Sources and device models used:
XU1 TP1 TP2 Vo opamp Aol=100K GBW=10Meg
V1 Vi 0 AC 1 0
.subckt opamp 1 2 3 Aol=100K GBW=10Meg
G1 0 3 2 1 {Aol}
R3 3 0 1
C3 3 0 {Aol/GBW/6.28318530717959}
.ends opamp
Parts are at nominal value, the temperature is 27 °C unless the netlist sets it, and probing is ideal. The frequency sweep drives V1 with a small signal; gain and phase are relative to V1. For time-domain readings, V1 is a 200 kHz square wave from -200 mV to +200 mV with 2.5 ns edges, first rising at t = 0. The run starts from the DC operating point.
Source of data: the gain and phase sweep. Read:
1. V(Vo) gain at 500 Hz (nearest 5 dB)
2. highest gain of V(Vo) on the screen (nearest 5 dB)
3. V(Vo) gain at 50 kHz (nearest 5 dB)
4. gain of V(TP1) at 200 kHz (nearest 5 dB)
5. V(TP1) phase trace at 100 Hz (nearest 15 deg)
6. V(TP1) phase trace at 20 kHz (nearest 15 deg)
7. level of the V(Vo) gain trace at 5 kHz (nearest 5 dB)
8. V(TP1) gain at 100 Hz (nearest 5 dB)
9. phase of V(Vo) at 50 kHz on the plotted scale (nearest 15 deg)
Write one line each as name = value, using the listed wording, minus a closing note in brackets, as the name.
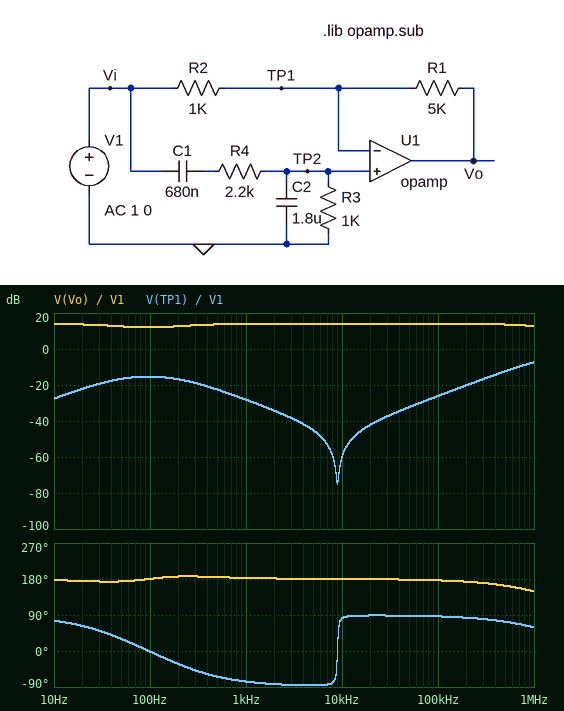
V(Vo) gain at 500 Hz = 15 dB
highest gain of V(Vo) on the screen = 15 dB
V(Vo) gain at 50 kHz = 15 dB
gain of V(TP1) at 200 kHz = -20 dB
V(TP1) phase trace at 100 Hz = 0 deg
V(TP1) phase trace at 20 kHz = 90 deg
level of the V(Vo) gain trace at 5 kHz = 15 dB
V(TP1) gain at 100 Hz = -15 dB
phase of V(Vo) at 50 kHz on the plotted scale = 180 deg
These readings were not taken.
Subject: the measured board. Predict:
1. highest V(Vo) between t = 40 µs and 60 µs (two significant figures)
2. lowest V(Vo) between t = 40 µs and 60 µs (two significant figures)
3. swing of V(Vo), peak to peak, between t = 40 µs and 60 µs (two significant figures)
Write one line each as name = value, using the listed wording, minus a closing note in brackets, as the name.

highest V(Vo) between t = 40 µs and 60 µs = 1.0 V
lowest V(Vo) between t = 40 µs and 60 µs = -990 mV
swing of V(Vo), peak to peak, between t = 40 µs and 60 µs = 2.0 V
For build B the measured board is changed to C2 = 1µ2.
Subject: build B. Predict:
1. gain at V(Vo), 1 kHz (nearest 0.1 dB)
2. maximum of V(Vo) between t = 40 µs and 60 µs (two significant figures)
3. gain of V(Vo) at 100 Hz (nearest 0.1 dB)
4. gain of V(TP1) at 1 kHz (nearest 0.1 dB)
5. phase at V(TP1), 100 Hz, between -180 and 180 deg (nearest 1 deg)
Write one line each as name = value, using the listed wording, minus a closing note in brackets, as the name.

gain at V(Vo), 1 kHz = 13.8 dB
maximum of V(Vo) between t = 40 µs and 60 µs = 1.0 V
gain of V(Vo) at 100 Hz = 11.6 dB
gain of V(TP1) at 1 kHz = -24.7 dB
phase at V(TP1), 100 Hz, between -180 and 180 deg = 8 deg
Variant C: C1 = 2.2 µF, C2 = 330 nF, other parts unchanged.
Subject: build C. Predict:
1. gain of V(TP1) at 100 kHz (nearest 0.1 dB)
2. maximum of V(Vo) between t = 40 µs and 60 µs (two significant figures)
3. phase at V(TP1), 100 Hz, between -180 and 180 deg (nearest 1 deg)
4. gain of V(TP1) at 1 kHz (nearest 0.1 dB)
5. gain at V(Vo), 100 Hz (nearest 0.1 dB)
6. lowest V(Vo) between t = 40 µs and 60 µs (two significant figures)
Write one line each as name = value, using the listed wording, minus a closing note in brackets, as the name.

gain of V(TP1) at 100 kHz = -26.4 dB
maximum of V(Vo) between t = 40 µs and 60 µs = 1.1 V
phase at V(TP1), 100 Hz, between -180 and 180 deg = 5 deg
gain of V(TP1) at 1 kHz = -15.0 dB
gain at V(Vo), 100 Hz = 10.2 dB
lowest V(Vo) between t = 40 µs and 60 µs = -940 mV
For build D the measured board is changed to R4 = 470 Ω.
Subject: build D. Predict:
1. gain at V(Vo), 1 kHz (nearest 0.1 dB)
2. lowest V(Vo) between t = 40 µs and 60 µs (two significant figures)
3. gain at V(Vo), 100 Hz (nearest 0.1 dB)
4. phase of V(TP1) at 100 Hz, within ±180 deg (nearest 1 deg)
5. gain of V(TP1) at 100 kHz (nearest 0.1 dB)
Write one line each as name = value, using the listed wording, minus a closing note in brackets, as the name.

gain at V(Vo), 1 kHz = 13.0 dB
lowest V(Vo) between t = 40 µs and 60 µs = -950 mV
gain at V(Vo), 100 Hz = 11.6 dB
phase of V(TP1) at 100 Hz, within ±180 deg = 24 deg
gain of V(TP1) at 100 kHz = -26.4 dB
